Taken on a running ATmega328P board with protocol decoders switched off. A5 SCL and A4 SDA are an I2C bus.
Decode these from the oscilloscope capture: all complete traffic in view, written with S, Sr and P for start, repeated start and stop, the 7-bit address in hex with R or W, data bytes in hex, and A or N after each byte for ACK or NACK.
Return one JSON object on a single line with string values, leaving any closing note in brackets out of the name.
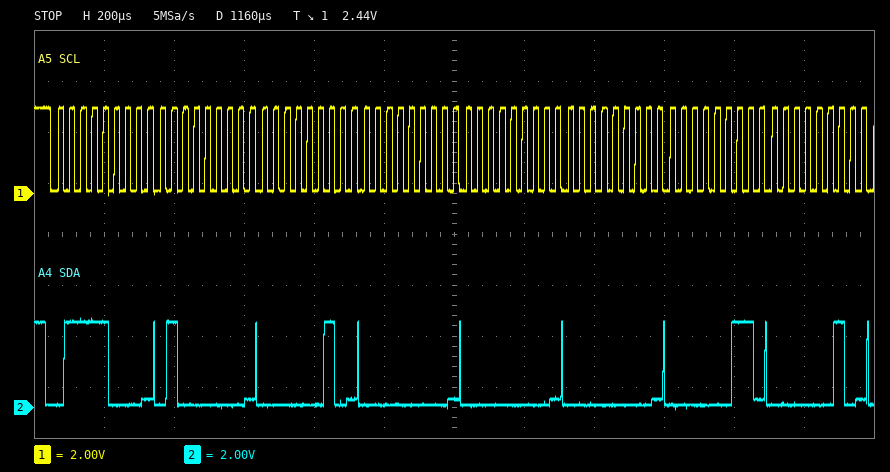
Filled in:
{"all complete traffic in view, written with S, Sr and P for start, repeated start and stop, the 7-bit address in hex with R or W, data bytes in hex, and A or N after each byte for ACK or NACK": "S 3CW A 40 A 02 A 00 A 00 A 00 A 03 A 02 A"}
